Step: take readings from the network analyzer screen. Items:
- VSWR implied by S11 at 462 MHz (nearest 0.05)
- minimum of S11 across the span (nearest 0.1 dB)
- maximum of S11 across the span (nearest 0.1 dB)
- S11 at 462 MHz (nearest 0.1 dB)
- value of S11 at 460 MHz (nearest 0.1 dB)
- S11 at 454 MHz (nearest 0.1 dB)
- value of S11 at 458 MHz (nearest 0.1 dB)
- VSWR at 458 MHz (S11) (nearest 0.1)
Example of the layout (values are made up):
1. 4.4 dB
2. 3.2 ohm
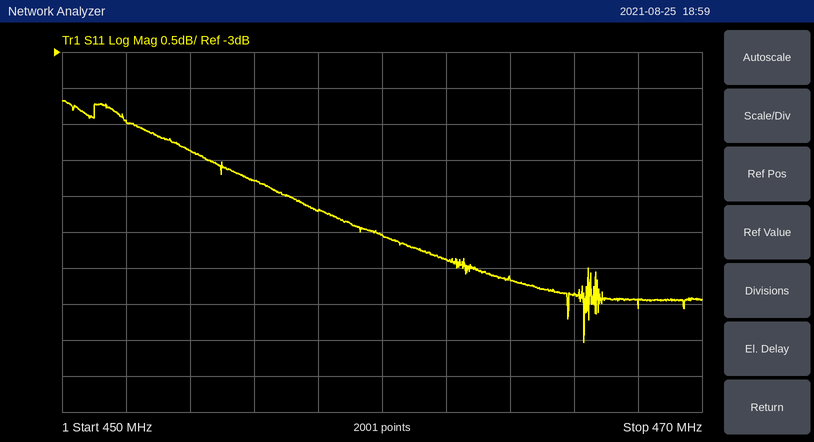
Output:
1. 3.05
2. -7.0 dB
3. -3.7 dB
4. -5.9 dB
5. -5.5 dB
6. -4.4 dB
7. -5.2 dB
8. 3.4
